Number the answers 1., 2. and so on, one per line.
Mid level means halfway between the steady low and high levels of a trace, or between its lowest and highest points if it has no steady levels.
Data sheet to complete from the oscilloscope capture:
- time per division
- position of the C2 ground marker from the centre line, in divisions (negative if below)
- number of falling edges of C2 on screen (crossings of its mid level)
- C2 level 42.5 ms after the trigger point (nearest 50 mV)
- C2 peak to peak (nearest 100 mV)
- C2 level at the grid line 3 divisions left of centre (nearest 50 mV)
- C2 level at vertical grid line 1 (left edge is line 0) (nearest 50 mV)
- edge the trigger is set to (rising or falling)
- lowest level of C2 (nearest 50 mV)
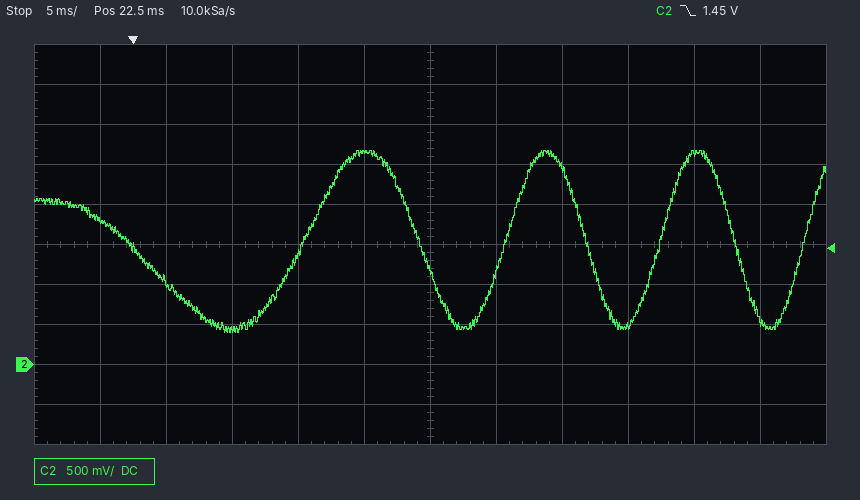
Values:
1. 5 ms
2. -3.0 div
3. 4
4. 2.65 V
5. 2.30 V
6. 450 mV
7. 1.80 V
8. falling
9. 400 mV
